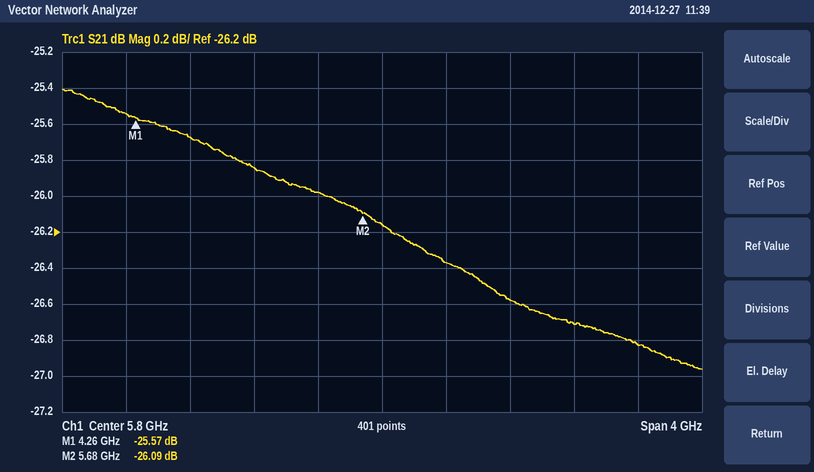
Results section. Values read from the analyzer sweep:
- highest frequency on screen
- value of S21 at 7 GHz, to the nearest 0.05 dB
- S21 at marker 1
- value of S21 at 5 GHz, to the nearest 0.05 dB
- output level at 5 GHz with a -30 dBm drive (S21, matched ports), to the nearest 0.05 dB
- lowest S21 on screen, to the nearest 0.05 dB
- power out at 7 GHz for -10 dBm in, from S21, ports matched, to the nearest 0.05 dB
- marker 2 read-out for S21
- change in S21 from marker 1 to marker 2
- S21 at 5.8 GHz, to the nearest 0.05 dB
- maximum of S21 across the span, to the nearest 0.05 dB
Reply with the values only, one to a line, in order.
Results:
7.8 GHz
-26.70 dB
-25.57 dB
-25.85 dB
-55.85 dBm
-26.95 dB
-36.70 dBm
-26.09 dB
-0.52 dB
-26.15 dB
-25.40 dB
